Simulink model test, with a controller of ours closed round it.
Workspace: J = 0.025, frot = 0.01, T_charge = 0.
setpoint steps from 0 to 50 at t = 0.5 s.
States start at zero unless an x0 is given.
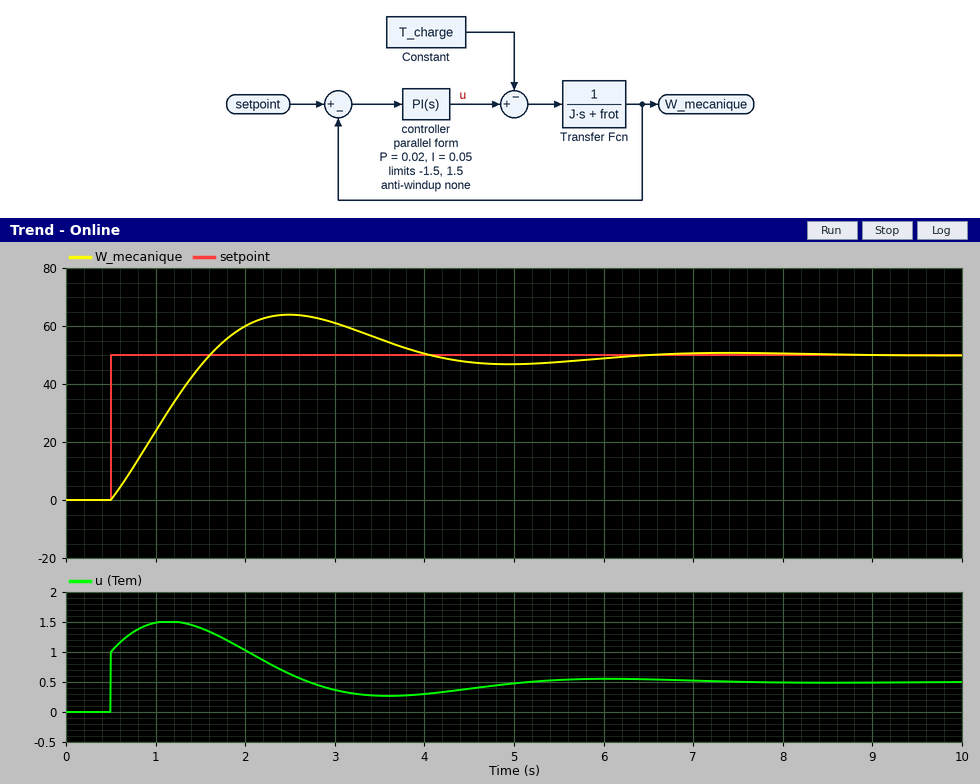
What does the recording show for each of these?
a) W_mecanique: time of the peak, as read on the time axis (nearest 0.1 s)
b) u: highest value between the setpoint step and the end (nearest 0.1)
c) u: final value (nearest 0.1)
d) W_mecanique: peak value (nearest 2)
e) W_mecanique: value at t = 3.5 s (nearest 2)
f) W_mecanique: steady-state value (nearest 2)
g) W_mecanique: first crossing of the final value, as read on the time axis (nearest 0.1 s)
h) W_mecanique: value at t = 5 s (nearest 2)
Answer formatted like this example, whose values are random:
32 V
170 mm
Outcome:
2.5 s
1.5
0.5
64
56
50
1.6 s
46
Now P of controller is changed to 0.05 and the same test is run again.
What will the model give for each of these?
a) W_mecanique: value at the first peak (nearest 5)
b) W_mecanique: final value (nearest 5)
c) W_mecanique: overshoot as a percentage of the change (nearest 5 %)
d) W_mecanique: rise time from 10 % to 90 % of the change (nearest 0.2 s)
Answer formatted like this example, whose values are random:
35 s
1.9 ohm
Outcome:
60
50
15 %
0.8 s
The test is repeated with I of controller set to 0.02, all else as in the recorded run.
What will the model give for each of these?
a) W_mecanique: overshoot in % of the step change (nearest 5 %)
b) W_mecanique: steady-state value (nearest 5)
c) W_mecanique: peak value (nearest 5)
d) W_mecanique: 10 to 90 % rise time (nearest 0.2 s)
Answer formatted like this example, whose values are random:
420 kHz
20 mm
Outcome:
10 %
50
55
1.4 s
